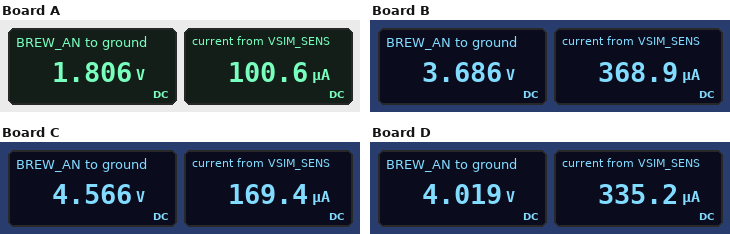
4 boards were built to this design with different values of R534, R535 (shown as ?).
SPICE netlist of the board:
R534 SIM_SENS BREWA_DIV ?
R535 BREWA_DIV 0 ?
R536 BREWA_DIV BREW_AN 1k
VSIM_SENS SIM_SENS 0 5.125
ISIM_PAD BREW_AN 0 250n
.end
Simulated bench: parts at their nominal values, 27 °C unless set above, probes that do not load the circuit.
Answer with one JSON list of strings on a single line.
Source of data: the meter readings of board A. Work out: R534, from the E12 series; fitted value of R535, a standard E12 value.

["33 kΩ", "18 kΩ"]
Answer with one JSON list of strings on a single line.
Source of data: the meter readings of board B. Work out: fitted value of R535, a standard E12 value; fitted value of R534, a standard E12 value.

["10 kΩ", "3.9 kΩ"]
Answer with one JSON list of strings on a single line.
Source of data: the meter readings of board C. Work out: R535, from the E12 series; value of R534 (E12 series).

["27 kΩ", "3.3 kΩ"]
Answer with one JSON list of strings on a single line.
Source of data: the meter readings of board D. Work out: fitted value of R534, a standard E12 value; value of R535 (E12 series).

["3.3 kΩ", "12 kΩ"]
